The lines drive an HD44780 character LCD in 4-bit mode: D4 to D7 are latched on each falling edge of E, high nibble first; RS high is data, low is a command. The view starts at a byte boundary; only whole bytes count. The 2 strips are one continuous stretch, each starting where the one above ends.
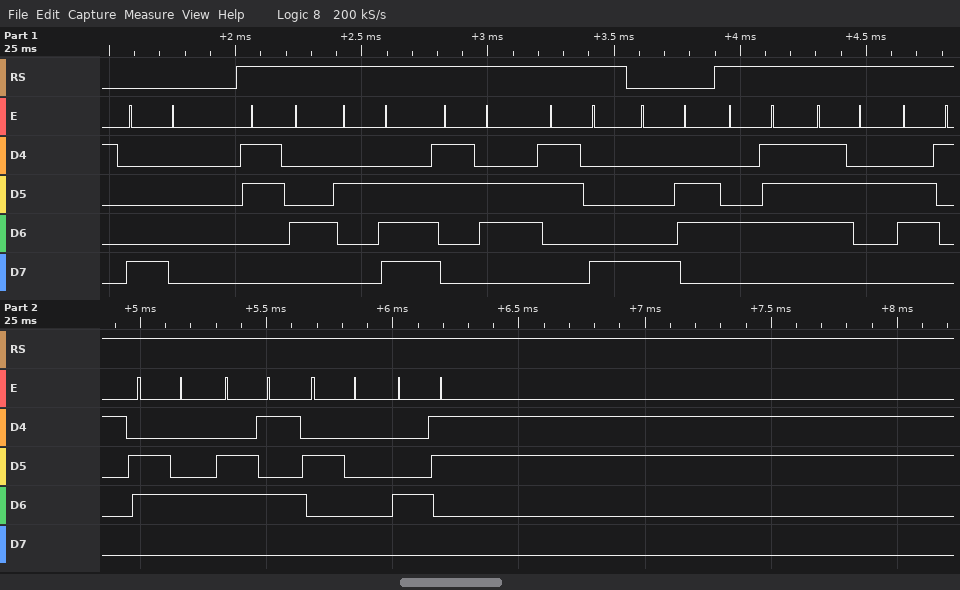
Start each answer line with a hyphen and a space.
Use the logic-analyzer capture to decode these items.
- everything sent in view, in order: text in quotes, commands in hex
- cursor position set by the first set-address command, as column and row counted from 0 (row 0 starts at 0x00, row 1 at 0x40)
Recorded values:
- 0x80 "4.68" 0x86 "Grade C"
- column 0, row 0
